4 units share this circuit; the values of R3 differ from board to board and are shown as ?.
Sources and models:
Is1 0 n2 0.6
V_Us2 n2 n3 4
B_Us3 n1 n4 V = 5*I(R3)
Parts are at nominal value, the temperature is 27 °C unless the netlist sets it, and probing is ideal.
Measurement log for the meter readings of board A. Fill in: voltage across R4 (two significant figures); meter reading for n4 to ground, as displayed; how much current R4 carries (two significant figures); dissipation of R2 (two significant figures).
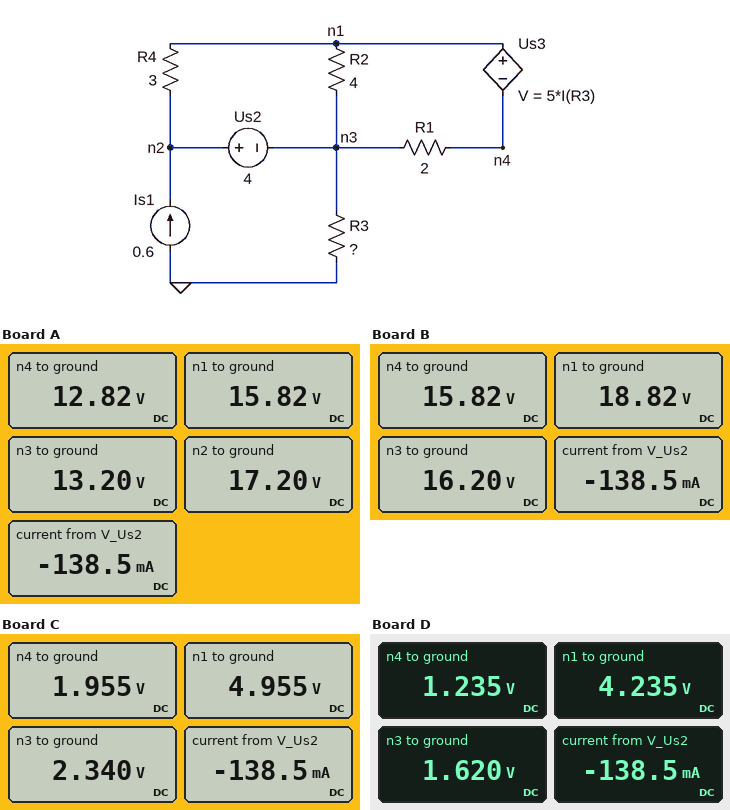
1.4 V
12.82 V
460 mA
1.7 W
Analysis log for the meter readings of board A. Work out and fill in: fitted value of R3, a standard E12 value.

22 Ω
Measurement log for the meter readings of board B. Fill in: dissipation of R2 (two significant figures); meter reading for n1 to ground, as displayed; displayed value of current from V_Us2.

1.7 W
18.82 V
-138.5 mA
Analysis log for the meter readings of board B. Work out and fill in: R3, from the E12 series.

27 Ω
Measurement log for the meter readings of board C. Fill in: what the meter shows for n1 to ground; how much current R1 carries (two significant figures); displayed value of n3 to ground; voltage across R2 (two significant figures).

4.955 V
190 mA
2.340 V
2.6 V
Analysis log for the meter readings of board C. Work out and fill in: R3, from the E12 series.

3.9 Ω
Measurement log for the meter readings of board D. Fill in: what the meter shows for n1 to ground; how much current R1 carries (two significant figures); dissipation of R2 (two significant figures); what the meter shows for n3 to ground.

4.235 V
190 mA
1.7 W
1.620 V
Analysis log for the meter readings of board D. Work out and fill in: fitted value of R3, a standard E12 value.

2.7 Ω
